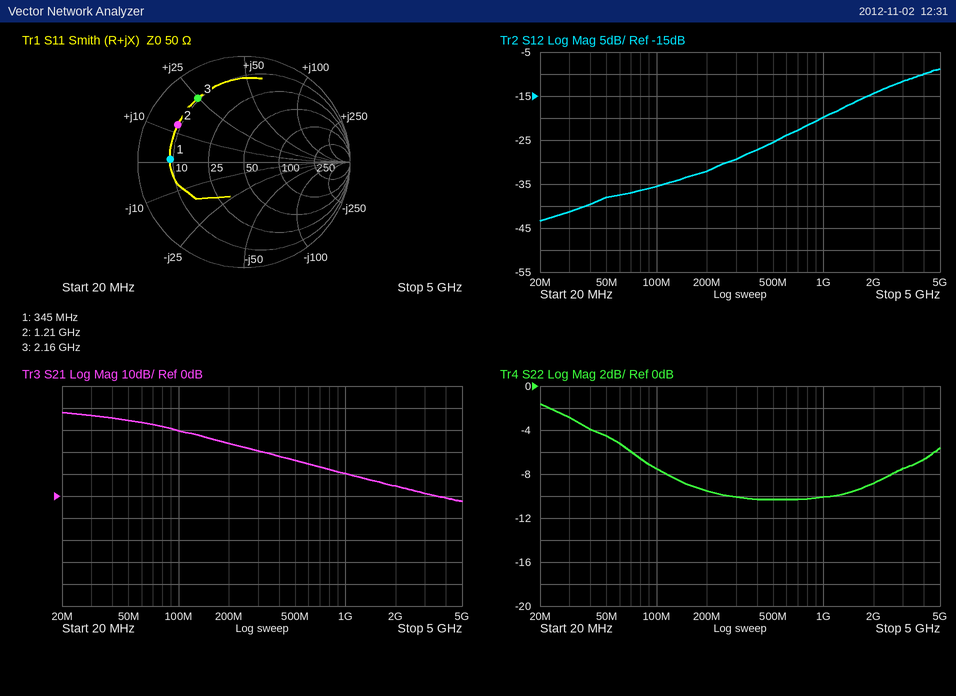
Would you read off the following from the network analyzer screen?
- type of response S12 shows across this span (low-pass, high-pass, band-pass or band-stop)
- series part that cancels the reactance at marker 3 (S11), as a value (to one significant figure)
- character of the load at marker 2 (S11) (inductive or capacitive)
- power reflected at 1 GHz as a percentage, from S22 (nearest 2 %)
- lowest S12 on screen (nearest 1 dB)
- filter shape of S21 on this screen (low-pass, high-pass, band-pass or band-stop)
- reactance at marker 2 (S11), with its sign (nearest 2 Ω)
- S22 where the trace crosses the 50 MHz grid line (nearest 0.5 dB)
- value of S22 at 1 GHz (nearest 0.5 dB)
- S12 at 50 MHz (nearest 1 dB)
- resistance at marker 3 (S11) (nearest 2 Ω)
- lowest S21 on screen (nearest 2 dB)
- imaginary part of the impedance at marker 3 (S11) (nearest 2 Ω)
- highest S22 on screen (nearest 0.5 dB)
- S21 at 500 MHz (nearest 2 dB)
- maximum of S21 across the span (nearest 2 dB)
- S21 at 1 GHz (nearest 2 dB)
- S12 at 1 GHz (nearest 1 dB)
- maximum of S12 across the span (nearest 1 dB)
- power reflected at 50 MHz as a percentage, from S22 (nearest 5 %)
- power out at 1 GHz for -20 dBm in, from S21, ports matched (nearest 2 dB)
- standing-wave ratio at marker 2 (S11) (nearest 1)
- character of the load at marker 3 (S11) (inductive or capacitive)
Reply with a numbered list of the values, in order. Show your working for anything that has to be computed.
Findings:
1. high-pass
2. C = 1/(2π × 2.16 GHz × 24 Ω) ≈ 3 pF
3. inductive
4. 10^(-10/10) ≈ 10 %
5. -43 dB
6. low-pass
7. +12 Ω
8. -4.5 dB
9. -10.0 dB
10. -38 dB
11. 10 Ω
12. -2 dB
13. +24 Ω
14. -1.5 dB
15. 16 dB
16. 38 dB
17. 10 dB
18. -20 dB
19. -9 dB
20. 10^(-4.5/10) ≈ 35 %
21. -20 dBm + (10 dB) = -10 dBm
22. 6
23. inductive
